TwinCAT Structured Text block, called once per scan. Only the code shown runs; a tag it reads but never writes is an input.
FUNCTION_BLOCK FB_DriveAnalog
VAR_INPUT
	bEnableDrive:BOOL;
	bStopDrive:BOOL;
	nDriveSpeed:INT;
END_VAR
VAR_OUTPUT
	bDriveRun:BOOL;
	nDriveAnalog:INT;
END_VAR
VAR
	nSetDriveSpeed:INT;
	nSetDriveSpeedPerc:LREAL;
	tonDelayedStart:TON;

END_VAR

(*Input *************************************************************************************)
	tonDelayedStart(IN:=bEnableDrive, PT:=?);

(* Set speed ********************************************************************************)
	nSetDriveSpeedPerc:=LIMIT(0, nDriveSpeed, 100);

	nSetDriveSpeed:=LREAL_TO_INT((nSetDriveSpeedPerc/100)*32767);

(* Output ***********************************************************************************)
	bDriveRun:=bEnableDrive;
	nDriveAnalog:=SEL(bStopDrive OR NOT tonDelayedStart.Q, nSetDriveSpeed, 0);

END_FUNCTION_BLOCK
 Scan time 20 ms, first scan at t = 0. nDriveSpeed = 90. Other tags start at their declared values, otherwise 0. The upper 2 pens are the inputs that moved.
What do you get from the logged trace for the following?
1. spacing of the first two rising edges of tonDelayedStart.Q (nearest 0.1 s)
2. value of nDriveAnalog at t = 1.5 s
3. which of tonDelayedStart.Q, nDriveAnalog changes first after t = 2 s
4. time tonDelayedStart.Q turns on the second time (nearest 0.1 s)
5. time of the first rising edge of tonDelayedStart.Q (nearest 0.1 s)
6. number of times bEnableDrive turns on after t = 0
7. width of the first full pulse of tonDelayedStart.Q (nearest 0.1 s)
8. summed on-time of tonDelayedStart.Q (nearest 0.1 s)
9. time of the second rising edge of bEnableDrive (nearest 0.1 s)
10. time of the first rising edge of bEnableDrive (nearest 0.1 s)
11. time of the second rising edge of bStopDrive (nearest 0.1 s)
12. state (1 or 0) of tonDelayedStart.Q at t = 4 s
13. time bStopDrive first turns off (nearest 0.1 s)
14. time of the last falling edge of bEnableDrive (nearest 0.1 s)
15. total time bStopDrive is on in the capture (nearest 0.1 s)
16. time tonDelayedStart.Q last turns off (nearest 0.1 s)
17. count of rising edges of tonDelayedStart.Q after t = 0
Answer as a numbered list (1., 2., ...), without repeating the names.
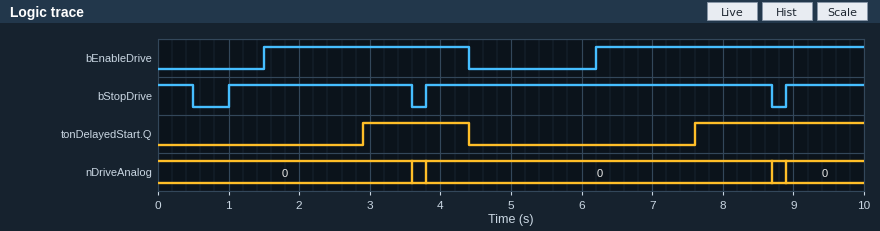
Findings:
1. 4.7 s
2. 0
3. tonDelayedStart.Q
4. 7.6 s
5. 2.9 s
6. 2
7. 1.5 s
8. 3.9 s
9. 6.2 s
10. 1.5 s
11. 3.8 s
12. 1
13. 0.5 s
14. 4.4 s
15. 9.1 s
16. 4.4 s
17. 2
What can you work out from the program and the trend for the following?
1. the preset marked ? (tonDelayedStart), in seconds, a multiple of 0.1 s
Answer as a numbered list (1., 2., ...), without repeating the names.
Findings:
1. 1.4 s
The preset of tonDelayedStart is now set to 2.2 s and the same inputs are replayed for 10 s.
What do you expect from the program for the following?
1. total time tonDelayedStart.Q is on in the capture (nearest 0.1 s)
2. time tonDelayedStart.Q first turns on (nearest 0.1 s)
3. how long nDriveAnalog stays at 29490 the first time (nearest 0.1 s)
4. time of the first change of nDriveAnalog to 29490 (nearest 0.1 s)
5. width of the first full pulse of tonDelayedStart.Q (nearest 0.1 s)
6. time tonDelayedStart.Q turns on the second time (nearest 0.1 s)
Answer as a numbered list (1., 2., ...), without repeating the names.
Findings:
1. 2.3 s
2. 3.7 s
3. 0.1 s
4. 3.7 s
5. 0.7 s
6. 8.4 s
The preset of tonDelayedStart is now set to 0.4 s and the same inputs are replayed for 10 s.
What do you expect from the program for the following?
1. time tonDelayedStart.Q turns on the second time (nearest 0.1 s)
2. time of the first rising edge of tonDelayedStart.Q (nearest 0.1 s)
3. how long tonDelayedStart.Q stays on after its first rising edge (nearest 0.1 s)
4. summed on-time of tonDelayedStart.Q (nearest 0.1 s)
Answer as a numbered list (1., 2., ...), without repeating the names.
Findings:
1. 6.6 s
2. 1.9 s
3. 2.5 s
4. 5.9 s
